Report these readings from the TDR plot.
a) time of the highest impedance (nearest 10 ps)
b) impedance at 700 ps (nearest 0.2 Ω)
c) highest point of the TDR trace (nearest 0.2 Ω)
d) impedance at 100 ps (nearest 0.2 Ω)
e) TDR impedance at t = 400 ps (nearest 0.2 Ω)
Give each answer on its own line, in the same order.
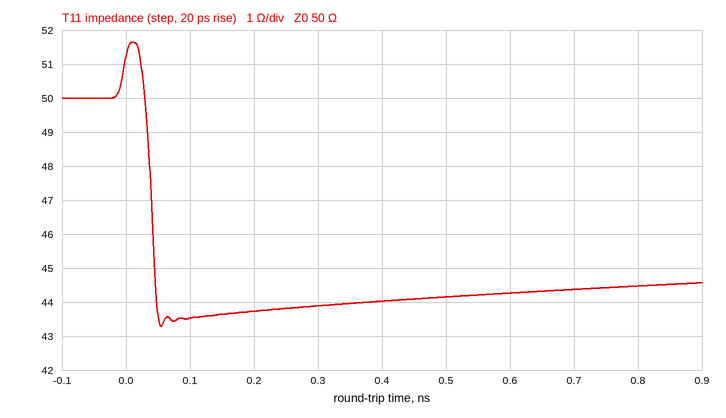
10 ps
44.4 Ω
51.6 Ω
43.6 Ω
44.0 Ω
